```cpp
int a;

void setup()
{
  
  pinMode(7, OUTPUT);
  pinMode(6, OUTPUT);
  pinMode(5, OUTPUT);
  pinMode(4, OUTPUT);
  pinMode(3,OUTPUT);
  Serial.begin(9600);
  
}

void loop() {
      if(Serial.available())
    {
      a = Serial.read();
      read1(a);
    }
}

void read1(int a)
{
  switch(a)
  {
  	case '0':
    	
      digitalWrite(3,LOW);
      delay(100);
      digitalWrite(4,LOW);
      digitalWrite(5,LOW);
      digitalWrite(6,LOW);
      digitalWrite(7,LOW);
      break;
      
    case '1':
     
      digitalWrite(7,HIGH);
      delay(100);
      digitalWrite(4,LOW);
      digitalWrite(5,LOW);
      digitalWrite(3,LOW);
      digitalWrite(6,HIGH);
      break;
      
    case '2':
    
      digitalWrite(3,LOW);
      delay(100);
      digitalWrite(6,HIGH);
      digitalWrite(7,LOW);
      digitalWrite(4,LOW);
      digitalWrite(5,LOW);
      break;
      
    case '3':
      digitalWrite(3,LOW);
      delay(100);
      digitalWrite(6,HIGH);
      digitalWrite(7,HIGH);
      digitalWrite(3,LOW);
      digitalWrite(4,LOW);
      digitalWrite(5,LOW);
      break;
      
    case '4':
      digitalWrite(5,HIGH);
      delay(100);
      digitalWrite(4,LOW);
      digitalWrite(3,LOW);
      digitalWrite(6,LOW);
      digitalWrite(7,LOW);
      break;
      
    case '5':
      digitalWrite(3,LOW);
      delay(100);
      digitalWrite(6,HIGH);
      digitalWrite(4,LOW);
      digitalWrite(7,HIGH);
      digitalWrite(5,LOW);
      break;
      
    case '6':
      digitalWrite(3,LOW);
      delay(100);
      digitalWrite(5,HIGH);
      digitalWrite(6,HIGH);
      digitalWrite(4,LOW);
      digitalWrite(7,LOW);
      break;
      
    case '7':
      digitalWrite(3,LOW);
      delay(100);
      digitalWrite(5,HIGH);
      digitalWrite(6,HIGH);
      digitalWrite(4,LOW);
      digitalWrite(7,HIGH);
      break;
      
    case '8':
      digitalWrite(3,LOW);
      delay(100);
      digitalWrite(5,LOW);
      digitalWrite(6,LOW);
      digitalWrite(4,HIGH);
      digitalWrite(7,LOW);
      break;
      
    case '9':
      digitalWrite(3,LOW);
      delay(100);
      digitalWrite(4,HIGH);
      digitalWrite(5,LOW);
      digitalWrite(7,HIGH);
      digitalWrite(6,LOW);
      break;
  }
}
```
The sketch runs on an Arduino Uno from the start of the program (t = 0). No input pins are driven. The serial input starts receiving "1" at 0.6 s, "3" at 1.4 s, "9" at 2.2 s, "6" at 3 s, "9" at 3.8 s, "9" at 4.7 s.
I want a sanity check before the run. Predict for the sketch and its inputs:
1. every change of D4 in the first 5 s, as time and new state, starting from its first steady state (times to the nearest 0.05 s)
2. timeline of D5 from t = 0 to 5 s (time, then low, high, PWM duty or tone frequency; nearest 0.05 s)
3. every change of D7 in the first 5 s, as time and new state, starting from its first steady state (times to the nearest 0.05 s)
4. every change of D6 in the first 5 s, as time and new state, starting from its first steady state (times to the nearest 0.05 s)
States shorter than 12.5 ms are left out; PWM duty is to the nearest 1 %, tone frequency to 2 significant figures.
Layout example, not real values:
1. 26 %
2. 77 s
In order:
1. 0 s low; 2.3 s high; 3.1 s low; 3.9 s high
2. 0 s low; 3.1 s high; 3.9 s low
3. 0 s low; 0.6 s high; 3.1 s low; 3.9 s high
4. 0 s low; 0.7 s high; 2.3 s low; 3.1 s high; 3.9 s low
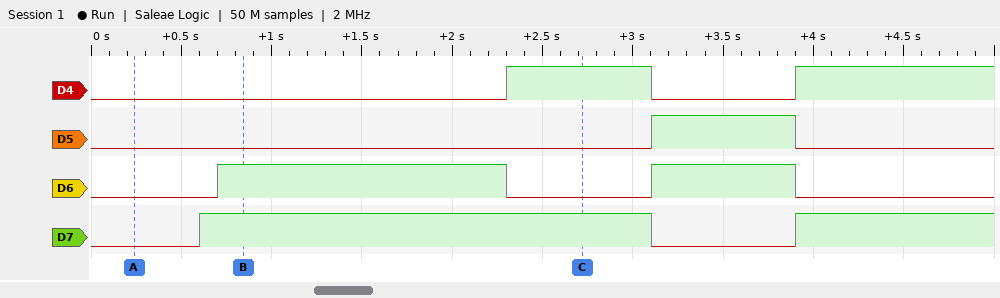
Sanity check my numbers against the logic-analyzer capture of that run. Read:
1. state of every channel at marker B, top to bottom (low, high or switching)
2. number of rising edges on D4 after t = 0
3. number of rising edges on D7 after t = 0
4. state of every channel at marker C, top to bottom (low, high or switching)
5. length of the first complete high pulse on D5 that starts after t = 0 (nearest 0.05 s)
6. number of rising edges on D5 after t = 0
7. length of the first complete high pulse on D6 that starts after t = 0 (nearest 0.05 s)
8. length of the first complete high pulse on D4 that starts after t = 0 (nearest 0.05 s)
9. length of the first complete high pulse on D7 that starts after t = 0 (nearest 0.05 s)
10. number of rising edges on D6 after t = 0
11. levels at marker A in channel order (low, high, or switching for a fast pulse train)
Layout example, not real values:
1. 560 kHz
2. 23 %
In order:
1. D4 low, D5 low, D6 high, D7 high
2. 2
3. 2
4. D4 high, D5 low, D6 low, D7 high
5. 0.80 s
6. 1
7. 1.60 s
8. 0.80 s
9. 2.50 s
10. 2
11. D4 low, D5 low, D6 low, D7 low
